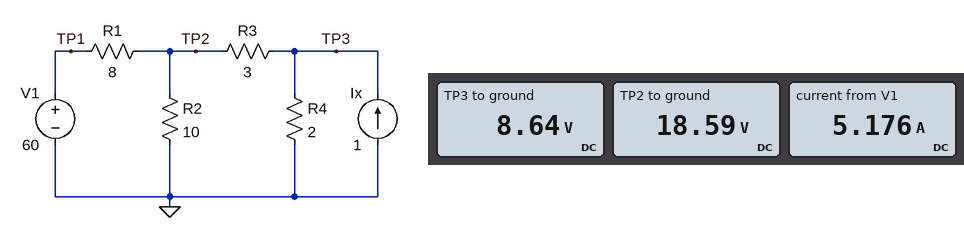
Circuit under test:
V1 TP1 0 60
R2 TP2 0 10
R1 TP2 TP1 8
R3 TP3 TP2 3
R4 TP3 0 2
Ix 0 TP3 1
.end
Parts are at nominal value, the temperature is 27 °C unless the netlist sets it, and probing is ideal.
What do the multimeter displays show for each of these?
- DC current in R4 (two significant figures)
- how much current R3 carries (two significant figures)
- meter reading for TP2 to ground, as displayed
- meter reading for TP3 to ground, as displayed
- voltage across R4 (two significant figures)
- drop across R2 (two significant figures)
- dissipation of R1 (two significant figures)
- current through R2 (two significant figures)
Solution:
4.3 A
3.3 A
18.59 V
8.64 V
8.6 V
19 V
210 W
1.9 A
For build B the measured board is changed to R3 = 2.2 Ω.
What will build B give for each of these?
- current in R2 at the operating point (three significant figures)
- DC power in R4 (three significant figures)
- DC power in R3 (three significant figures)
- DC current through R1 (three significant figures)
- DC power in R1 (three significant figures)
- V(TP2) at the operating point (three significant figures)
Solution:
1.72 A
42.8 W
28.9 W
5.35 A
229 W
17.2 V
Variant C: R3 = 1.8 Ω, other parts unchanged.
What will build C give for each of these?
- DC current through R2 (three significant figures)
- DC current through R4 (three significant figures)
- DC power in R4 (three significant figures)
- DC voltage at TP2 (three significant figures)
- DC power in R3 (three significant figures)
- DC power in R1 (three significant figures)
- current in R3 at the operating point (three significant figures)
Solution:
1.64 A
4.80 A
46.1 W
16.4 V
26.0 W
237 W
3.80 A
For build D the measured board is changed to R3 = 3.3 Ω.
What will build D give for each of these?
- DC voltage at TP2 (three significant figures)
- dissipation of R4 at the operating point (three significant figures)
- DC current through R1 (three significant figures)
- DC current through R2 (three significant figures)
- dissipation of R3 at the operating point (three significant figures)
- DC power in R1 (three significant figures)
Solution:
19.0 V
35.5 W
5.12 A
1.90 A
34.1 W
210 W
